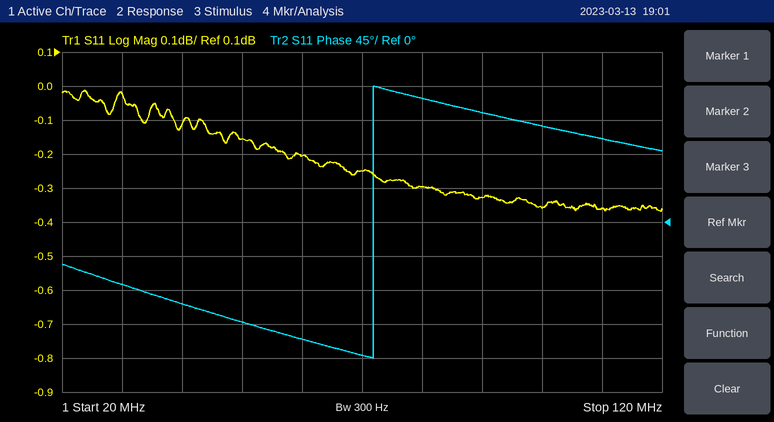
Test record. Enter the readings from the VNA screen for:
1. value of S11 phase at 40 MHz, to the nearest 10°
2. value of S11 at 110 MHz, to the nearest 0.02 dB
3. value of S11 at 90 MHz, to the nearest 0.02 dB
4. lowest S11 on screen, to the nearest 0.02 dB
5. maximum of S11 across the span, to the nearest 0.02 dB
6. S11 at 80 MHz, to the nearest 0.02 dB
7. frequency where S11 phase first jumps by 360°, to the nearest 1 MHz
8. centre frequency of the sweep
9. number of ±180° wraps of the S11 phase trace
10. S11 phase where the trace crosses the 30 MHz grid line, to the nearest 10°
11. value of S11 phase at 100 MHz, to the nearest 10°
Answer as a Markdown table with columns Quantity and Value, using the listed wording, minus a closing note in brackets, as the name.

| Quantity | Value |
|---|---|
| value of S11 phase at 40 MHz, to the nearest 10° | -110° |
| value of S11 at 110 MHz, to the nearest 0.02 dB | -0.36 dB |
| value of S11 at 90 MHz, to the nearest 0.02 dB | -0.32 dB |
| lowest S11 on screen, to the nearest 0.02 dB | -0.36 dB |
| maximum of S11 across the span, to the nearest 0.02 dB | -0.02 dB |
| S11 at 80 MHz, to the nearest 0.02 dB | -0.30 dB |
| frequency where S11 phase first jumps by 360°, to the nearest 1 MHz | 72 MHz |
| centre frequency of the sweep | 70 MHz |
| number of ±180° wraps of the S11 phase trace | 1 |
| S11 phase where the trace crosses the 30 MHz grid line, to the nearest 10° | -80° |
| value of S11 phase at 100 MHz, to the nearest 10° | 130° |
